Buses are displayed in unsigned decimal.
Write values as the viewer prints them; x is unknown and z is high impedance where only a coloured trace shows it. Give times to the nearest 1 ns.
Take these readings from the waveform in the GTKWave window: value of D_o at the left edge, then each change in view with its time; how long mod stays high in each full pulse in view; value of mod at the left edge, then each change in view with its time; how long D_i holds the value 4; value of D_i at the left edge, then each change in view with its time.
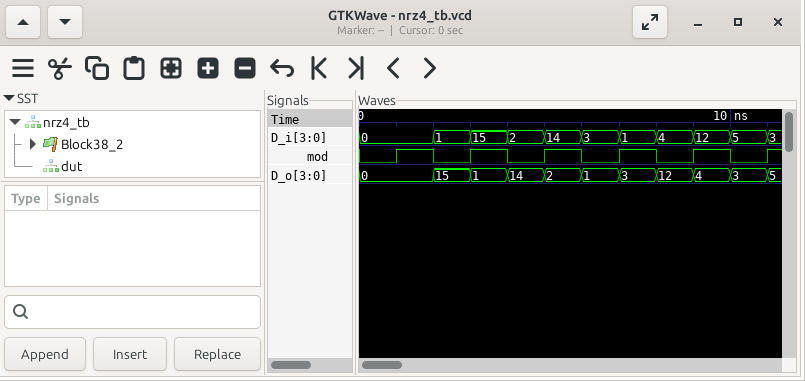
0, 15 at 2 ns, 1 at 3 ns, 14 at 4 ns, 2 at 5 ns, 1 at 6 ns, 3 at 7 ns, 12 at 8 ns, 4 at 9 ns, 3 at 10 ns, 5 at 11 ns
1 ns, 1 ns, 1 ns, 1 ns, 1 ns
0, 1 at 1 ns, 0 at 2 ns, 1 at 3 ns, 0 at 4 ns, 1 at 5 ns, 0 at 6 ns, 1 at 7 ns, 0 at 8 ns, 1 at 9 ns, 0 at 10 ns, 1 at 11 ns
1 ns
0, 1 at 2 ns, 15 at 3 ns, 2 at 4 ns, 14 at 5 ns, 3 at 6 ns, 1 at 7 ns, 4 at 8 ns, 12 at 9 ns, 5 at 10 ns, 3 at 11 ns
